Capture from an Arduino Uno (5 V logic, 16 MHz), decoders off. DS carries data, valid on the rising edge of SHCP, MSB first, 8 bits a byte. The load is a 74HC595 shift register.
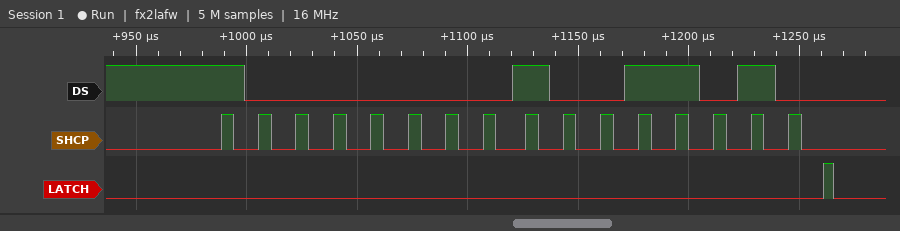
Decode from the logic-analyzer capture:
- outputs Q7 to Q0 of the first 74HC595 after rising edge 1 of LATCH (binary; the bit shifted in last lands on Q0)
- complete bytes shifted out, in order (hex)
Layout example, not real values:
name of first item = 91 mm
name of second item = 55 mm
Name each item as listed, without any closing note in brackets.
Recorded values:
outputs Q7 to Q0 of the first 74HC595 after rising edge 1 of LATCH = 10011010
complete bytes shifted out, in order = 80 9A
